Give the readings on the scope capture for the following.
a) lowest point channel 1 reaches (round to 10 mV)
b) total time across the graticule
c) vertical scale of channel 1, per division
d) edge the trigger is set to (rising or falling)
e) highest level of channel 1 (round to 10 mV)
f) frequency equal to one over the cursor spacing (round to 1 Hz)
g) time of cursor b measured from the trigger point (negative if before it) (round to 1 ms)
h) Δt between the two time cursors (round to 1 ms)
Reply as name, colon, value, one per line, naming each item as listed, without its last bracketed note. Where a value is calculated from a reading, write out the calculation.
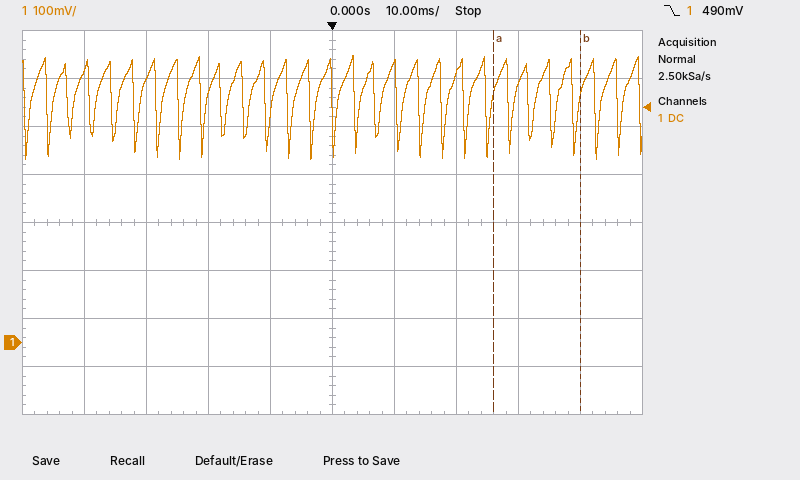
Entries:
lowest point channel 1 reaches: 380 mV
total time across the graticule: 100 ms
vertical scale of channel 1, per division: 100 mV
edge the trigger is set to: falling
highest level of channel 1: 600 mV
frequency equal to one over the cursor spacing: 1 / 14 ms ≈ 71 Hz
time of cursor b measured from the trigger point (negative if before it): +40 ms
Δt between the two time cursors: 14 ms
